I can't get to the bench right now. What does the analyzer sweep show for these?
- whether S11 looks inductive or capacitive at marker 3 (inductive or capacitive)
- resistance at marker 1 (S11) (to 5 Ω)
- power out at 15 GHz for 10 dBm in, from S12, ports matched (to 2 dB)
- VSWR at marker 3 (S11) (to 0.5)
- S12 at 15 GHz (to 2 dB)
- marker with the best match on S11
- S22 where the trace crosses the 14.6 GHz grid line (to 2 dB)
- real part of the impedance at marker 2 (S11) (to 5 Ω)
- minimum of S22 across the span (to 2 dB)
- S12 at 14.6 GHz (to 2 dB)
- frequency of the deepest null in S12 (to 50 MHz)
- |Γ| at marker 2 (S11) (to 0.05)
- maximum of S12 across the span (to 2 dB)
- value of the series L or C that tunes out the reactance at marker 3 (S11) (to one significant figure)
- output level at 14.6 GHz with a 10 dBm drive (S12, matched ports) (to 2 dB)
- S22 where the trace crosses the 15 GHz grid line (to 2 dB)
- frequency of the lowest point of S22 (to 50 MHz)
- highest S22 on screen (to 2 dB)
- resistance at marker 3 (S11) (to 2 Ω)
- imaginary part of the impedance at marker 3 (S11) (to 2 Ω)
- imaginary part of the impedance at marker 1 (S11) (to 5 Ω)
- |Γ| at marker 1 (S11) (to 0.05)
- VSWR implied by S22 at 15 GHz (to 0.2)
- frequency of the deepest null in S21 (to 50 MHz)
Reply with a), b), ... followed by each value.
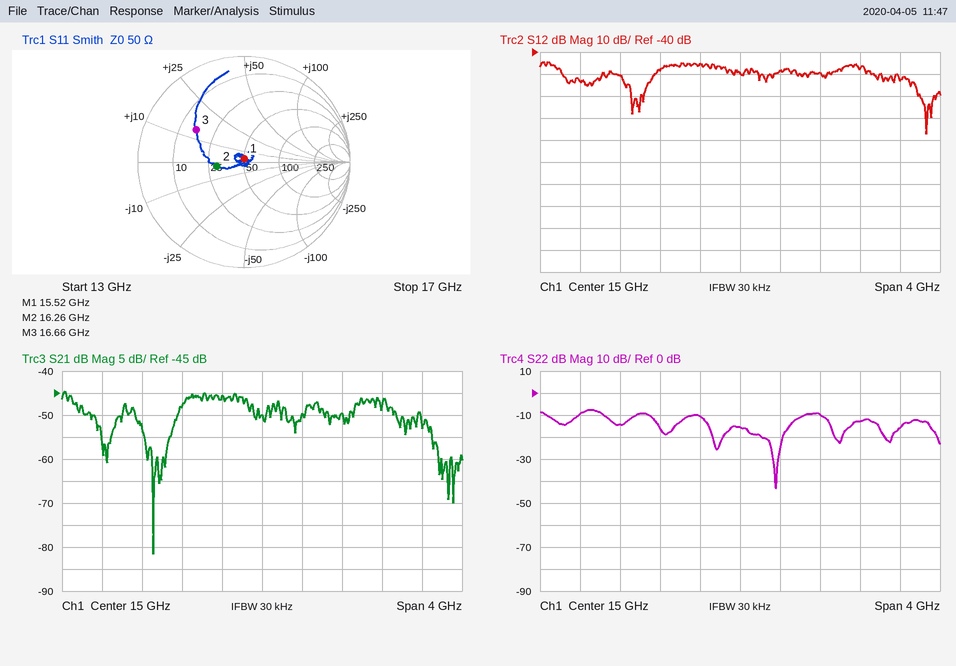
a) inductive
b) 50 Ω
c) -40 dBm
d) 3.5
e) -50 dB
f) marker 1
g) -10 dB
h) 30 Ω
i) -44 dB
j) -46 dB
k) 16.85 GHz
l) 0.25
m) -44 dB
n) 700 fF
o) -36 dBm
p) -16 dB
q) 15.35 GHz
r) -8 dB
s) 16 Ω
t) +14 Ω
u) +5 Ω
v) 0.05
w) 1.4
x) 13.90 GHz
